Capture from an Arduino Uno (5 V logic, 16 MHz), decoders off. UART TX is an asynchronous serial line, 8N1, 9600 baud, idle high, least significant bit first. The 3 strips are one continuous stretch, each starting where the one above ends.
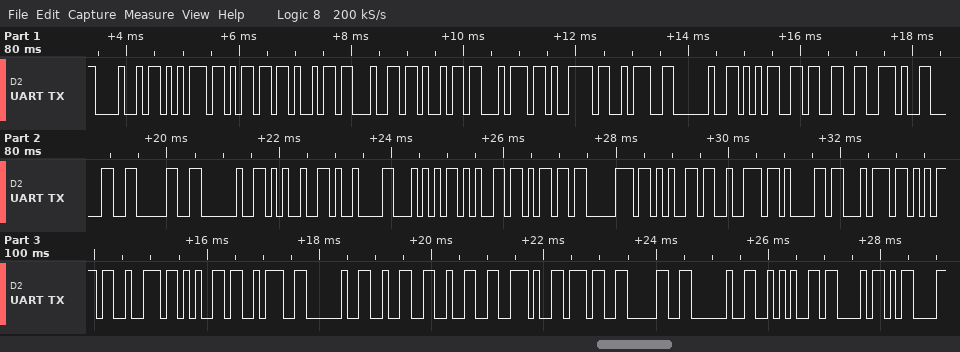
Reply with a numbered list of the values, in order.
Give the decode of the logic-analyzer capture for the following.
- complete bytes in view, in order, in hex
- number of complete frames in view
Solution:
1. 48 75 6D 69 64 69 74 79 3A 20 35 33 2E 30 30 20 25 09 54 65 6D 70 65 72 61 74 75 72 65 3A 20 32 32 2E 37 30 20 2A 43 0D
2. 40
